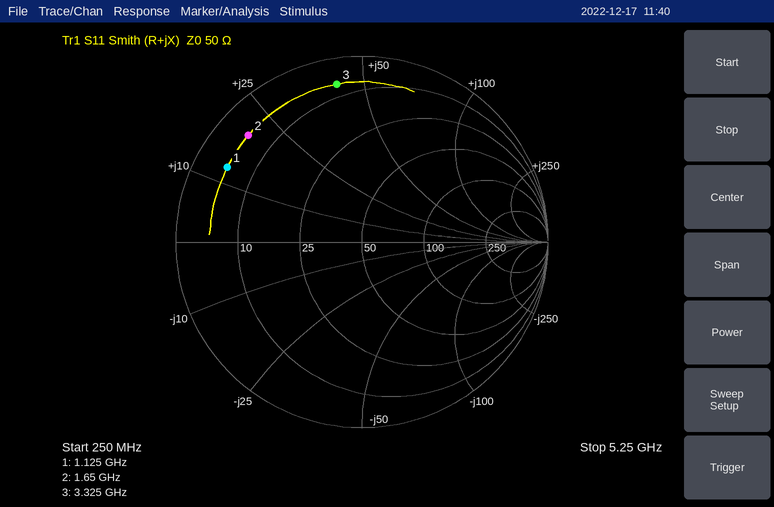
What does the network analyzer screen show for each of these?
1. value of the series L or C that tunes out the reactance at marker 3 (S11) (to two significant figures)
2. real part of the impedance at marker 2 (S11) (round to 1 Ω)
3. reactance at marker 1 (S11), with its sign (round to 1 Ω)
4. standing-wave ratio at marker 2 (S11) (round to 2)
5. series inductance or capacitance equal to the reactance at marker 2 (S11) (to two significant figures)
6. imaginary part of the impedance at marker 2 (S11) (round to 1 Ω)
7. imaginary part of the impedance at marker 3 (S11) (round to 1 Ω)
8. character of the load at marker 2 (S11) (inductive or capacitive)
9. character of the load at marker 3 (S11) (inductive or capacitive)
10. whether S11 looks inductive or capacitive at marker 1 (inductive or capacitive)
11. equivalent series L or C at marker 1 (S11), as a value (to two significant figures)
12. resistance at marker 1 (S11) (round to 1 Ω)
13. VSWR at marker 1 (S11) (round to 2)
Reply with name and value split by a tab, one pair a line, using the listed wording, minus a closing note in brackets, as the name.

value of the series L or C that tunes out the reactance at marker 3 (S11)	1.1 pF
real part of the impedance at marker 2 (S11)	5 Ω
reactance at marker 1 (S11), with its sign	+13 Ω
standing-wave ratio at marker 2 (S11)	12
series inductance or capacitance equal to the reactance at marker 2 (S11)	1.9 nH
imaginary part of the impedance at marker 2 (S11)	+20 Ω
imaginary part of the impedance at marker 3 (S11)	+42 Ω
character of the load at marker 2 (S11)	inductive
character of the load at marker 3 (S11)	inductive
whether S11 looks inductive or capacitive at marker 1	inductive
equivalent series L or C at marker 1 (S11), as a value	1.8 nH
resistance at marker 1 (S11)	5 Ω
VSWR at marker 1 (S11)	10
